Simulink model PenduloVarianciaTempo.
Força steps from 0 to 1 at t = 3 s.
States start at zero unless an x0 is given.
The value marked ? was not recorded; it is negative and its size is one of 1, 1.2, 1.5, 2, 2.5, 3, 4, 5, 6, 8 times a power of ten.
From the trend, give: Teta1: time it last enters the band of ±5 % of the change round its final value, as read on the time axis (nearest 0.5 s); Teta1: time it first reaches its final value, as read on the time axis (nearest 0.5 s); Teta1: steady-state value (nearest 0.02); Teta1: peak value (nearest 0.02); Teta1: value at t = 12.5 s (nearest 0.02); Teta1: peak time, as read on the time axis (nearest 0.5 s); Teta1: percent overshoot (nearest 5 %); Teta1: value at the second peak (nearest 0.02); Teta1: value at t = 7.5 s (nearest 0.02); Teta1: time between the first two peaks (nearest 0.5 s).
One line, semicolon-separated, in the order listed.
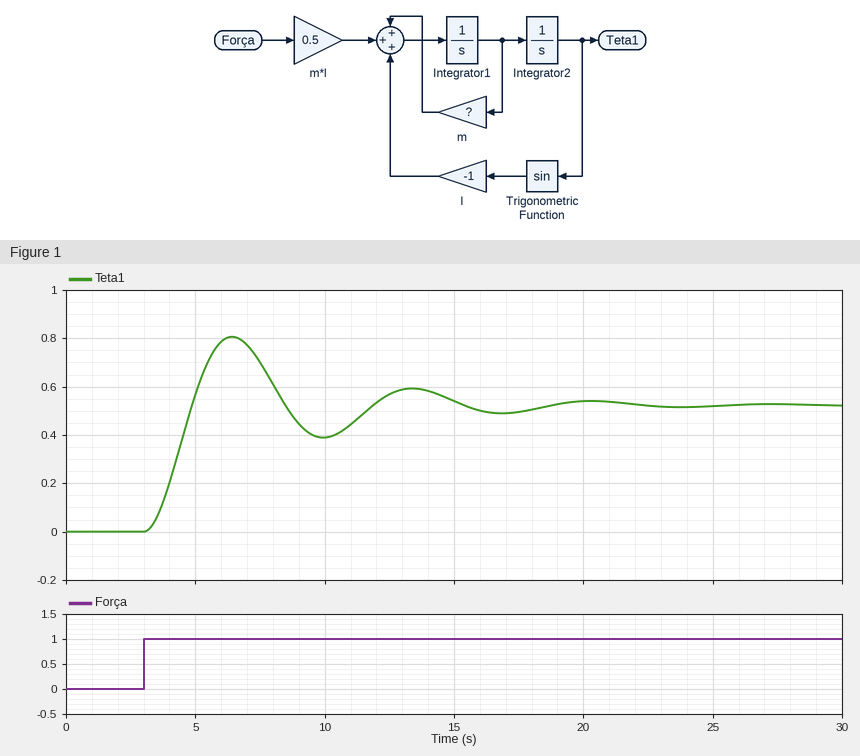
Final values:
17.5 s; 5.0 s; 0.52; 0.80; 0.56; 6.5 s; 55 %; 0.60; 0.70; 7.0 s
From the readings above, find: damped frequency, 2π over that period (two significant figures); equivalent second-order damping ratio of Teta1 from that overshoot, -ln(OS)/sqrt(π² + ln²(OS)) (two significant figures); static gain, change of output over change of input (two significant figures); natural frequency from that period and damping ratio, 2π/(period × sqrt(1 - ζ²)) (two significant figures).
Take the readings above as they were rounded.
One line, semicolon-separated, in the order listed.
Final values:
0.90 rad/s; 0.19; 0.52; 0.91 rad/s
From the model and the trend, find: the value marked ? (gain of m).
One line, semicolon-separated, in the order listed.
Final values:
-0.4
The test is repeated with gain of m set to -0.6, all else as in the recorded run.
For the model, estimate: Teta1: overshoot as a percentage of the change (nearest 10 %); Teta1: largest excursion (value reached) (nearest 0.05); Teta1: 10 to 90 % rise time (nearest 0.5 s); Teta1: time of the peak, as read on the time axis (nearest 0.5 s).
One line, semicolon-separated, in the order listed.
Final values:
40 %; 0.70; 1.5 s; 6.5 s
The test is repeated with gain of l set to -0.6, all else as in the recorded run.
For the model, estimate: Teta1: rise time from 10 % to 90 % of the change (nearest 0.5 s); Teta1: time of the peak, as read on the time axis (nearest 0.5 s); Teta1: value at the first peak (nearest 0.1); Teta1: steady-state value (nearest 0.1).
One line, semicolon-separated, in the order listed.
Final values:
2.0 s; 8.5 s; 1.4; 1.0
